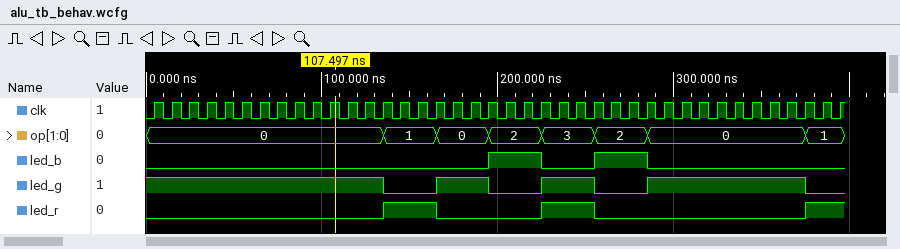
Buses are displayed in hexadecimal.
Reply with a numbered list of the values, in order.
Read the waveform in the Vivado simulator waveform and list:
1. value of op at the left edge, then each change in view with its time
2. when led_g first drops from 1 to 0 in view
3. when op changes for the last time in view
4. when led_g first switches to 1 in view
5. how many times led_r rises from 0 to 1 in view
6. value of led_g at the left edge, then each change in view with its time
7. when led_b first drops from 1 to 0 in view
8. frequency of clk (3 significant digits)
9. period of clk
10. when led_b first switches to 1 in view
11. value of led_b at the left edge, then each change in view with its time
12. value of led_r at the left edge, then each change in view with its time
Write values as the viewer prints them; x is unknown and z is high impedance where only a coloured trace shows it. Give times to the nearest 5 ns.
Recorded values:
1. 0, 1 at 135 ns, 0 at 165 ns, 2 at 195 ns, 3 at 225 ns, 2 at 255 ns, 0 at 285 ns, 1 at 375 ns
2. 135 ns
3. 375 ns
4. 165 ns
5. 3
6. 1, 0 at 135 ns, 1 at 165 ns, 0 at 195 ns, 1 at 225 ns, 0 at 255 ns, 1 at 285 ns, 0 at 375 ns
7. 225 ns
8. 100 MHz
9. 10 ns
10. 195 ns
11. 0, 1 at 195 ns, 0 at 225 ns, 1 at 255 ns, 0 at 285 ns
12. 0, 1 at 135 ns, 0 at 165 ns, 1 at 225 ns, 0 at 255 ns, 1 at 375 ns
